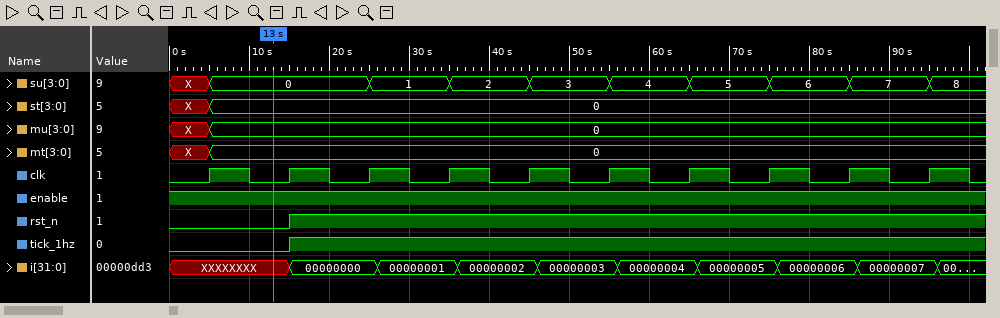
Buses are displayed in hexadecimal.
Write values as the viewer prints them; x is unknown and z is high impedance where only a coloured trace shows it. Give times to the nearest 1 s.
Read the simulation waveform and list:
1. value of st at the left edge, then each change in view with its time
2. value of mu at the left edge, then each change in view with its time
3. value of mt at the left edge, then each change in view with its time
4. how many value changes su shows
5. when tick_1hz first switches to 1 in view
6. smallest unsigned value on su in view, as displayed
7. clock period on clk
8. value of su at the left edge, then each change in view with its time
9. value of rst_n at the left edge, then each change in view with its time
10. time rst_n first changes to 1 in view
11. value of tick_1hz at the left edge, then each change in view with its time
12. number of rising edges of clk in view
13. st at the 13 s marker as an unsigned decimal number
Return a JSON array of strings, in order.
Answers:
["X, 0 at 5 s", "X, 0 at 5 s", "X, 0 at 5 s", "9", "15 s", "0", "10 s", "X, 0 at 5 s, 1 at 25 s, 2 at 35 s, 3 at 45 s, 4 at 55 s, 5 at 65 s, 6 at 75 s, 7 at 85 s, 8 at 95 s", "0, 1 at 15 s", "15 s", "0, 1 at 15 s", "10", "0"]
